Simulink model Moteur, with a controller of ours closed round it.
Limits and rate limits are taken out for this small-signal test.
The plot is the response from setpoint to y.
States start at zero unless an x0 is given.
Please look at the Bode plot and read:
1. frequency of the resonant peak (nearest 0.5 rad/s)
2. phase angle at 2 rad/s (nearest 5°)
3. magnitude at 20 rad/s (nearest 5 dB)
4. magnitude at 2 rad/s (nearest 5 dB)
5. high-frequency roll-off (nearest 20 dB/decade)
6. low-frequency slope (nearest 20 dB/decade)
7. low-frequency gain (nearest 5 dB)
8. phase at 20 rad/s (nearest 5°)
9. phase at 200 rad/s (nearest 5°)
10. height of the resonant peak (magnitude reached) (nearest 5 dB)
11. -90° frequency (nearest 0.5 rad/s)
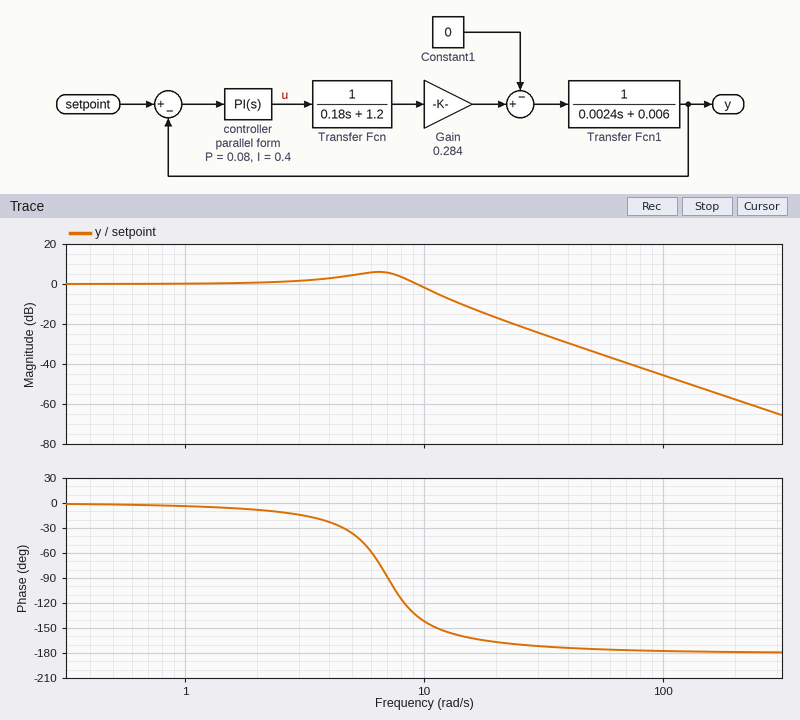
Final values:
6.5 rad/s
-10°
-15 dB
0 dB
-40 dB/decade
0 dB/decade
0 dB
-165°
-180°
5 dB
7.0 rad/s
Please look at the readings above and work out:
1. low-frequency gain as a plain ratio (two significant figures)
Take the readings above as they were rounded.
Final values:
1.0
